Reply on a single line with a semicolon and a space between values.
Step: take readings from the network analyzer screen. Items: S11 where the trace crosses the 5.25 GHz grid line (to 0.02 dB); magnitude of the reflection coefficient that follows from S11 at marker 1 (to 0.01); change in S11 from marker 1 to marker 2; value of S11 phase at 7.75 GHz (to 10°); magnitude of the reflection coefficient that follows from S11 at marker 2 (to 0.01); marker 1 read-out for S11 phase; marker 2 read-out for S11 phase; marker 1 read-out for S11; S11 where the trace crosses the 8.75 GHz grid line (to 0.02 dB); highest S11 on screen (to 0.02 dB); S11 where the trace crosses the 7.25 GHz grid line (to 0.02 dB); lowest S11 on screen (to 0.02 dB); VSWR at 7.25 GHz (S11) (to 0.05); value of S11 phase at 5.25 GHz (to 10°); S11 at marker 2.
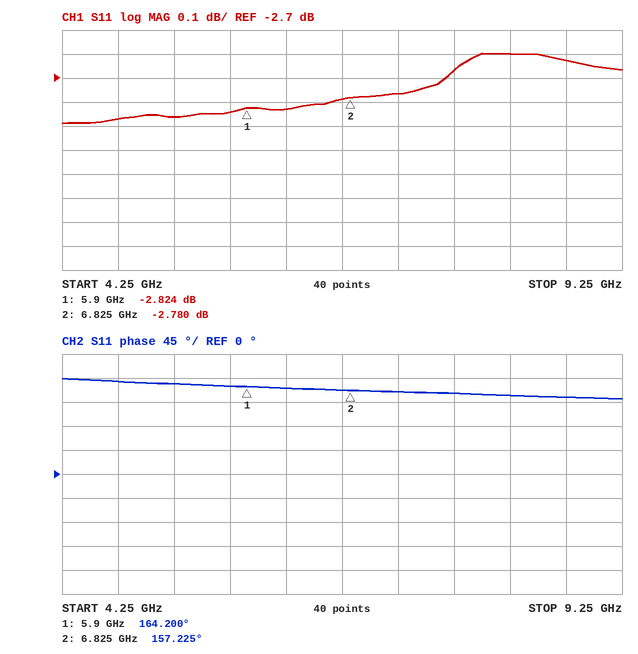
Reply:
-2.86 dB; 0.72; 0.044 dB; 150°; 0.73; 164.200°; 157.225°; -2.824 dB; -2.62 dB; -2.60 dB; -2.76 dB; -2.88 dB; 6.35; 170°; -2.780 dB
